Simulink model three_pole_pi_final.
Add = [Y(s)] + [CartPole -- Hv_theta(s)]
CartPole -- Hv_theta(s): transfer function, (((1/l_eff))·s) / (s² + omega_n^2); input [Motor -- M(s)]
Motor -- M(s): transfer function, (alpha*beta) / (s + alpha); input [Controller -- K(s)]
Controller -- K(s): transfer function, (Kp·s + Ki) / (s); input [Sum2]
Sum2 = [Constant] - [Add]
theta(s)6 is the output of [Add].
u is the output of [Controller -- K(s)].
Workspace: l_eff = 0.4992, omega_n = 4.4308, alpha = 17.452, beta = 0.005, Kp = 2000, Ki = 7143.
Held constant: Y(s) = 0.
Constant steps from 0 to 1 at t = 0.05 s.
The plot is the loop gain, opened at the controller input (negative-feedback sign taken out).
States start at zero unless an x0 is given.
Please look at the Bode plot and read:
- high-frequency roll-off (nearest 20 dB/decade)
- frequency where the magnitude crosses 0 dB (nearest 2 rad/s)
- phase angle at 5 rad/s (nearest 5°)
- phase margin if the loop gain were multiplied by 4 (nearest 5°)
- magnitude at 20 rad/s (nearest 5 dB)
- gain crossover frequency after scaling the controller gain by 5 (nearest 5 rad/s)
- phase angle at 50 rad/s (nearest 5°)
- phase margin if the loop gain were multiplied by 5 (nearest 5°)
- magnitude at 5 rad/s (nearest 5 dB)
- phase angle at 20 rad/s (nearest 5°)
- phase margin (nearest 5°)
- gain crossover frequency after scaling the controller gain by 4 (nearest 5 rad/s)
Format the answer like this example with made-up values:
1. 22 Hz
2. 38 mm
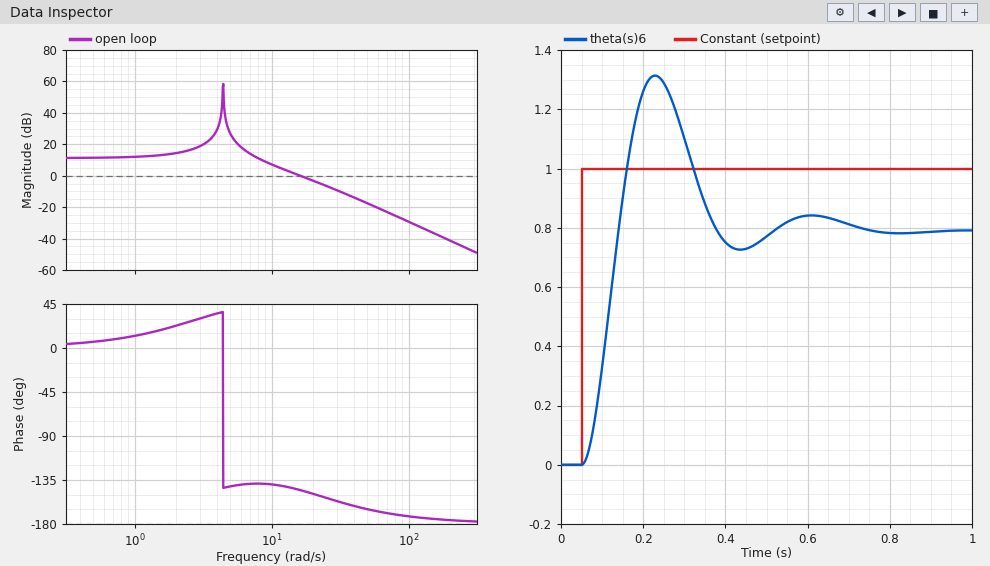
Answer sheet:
1. -40 dB/decade
2. 16 rad/s
3. -140°
4. 20°
5. -5 dB
6. 40 rad/s
7. -165°
8. 20°
9. 25 dB
10. -150°
11. 35°
12. 35 rad/s
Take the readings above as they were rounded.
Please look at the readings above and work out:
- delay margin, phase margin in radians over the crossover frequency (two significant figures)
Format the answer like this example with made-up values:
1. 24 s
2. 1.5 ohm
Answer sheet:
1. 0.038 s
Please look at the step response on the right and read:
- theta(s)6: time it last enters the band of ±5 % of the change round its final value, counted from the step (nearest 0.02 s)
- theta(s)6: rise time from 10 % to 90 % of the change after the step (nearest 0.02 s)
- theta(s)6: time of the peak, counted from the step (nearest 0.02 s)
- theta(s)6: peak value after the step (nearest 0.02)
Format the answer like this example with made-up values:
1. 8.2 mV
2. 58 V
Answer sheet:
1. 0.62 s
2. 0.06 s
3. 0.18 s
4. 1.32
